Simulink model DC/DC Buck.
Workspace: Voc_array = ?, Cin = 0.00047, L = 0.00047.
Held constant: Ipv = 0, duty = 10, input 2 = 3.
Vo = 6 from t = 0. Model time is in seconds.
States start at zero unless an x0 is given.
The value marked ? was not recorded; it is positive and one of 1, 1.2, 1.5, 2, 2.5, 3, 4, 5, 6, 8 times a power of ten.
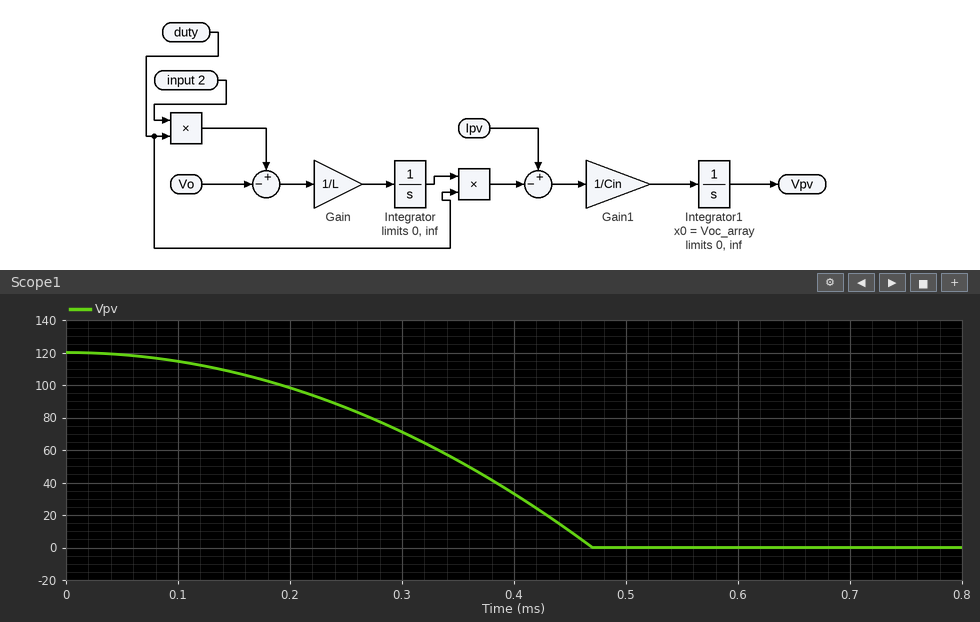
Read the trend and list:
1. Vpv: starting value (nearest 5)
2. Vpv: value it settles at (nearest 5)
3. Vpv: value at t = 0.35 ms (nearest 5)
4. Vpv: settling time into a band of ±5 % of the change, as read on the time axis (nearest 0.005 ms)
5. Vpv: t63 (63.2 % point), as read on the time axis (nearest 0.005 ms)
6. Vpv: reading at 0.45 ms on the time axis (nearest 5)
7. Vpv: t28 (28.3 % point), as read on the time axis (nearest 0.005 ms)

120
0
55
0.460 ms
0.375 ms
10
0.250 ms
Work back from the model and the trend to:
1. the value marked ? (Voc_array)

120
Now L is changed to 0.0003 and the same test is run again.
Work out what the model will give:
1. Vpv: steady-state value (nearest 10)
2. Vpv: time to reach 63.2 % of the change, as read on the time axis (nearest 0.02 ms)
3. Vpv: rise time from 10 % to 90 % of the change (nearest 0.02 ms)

0
0.30 ms
0.24 ms
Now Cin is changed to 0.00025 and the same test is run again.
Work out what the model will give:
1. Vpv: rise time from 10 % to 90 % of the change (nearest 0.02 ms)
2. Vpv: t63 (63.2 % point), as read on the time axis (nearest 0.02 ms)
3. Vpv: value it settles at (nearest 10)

0.22 ms
0.28 ms
0
